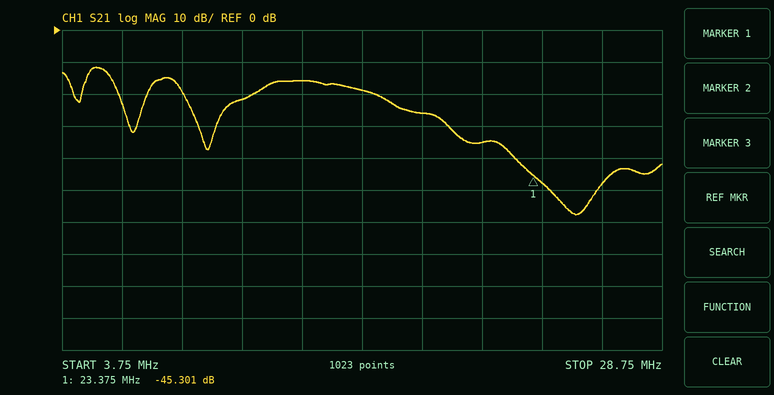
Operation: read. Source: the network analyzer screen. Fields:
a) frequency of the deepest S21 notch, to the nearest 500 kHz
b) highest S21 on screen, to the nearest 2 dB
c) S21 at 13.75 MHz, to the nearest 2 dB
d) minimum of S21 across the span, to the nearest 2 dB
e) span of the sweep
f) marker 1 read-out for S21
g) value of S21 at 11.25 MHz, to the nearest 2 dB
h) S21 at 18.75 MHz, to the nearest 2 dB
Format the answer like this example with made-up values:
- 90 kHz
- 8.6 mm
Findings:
- 25.0 MHz
- -12 dB
- -16 dB
- -58 dB
- 25 MHz
- -45.301 dB
- -22 dB
- -26 dB
